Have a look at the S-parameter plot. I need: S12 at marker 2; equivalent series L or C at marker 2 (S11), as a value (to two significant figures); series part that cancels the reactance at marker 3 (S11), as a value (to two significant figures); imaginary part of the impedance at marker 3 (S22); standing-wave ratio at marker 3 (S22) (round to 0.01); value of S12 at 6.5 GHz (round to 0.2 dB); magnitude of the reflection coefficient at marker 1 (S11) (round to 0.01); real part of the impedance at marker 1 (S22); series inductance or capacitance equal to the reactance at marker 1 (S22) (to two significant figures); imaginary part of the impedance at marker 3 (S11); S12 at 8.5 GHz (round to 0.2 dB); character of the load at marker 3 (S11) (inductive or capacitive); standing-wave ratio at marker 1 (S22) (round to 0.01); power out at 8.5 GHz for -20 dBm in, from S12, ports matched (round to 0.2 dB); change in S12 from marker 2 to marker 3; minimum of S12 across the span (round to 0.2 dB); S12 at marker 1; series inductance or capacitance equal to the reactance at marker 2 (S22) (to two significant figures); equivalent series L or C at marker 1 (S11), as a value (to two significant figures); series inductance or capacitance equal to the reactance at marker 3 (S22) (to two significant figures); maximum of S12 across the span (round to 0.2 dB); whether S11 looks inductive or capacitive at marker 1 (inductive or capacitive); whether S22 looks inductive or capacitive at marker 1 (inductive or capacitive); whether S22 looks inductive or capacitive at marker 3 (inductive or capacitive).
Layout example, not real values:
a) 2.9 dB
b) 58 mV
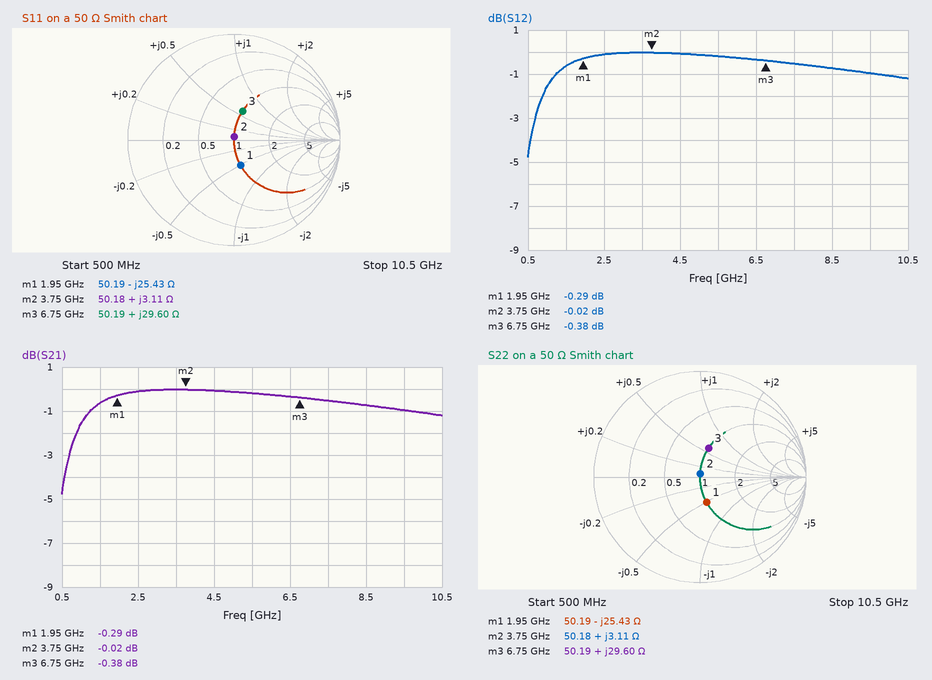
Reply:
a) -0.02 dB
b) 130 pH
c) 800 fF
d) +29.60 Ω
e) 1.79
f) -0.4 dB
g) 0.25
h) 50.19 Ω
i) 3.2 pF
j) +29.60 Ω
k) -0.8 dB
l) inductive
m) 1.65
n) -20.8 dBm
o) -0.36 dB
p) -4.8 dB
q) -0.29 dB
r) 130 pH
s) 3.2 pF
t) 700 pH
u) 0.0 dB
v) capacitive
w) capacitive
x) inductive
